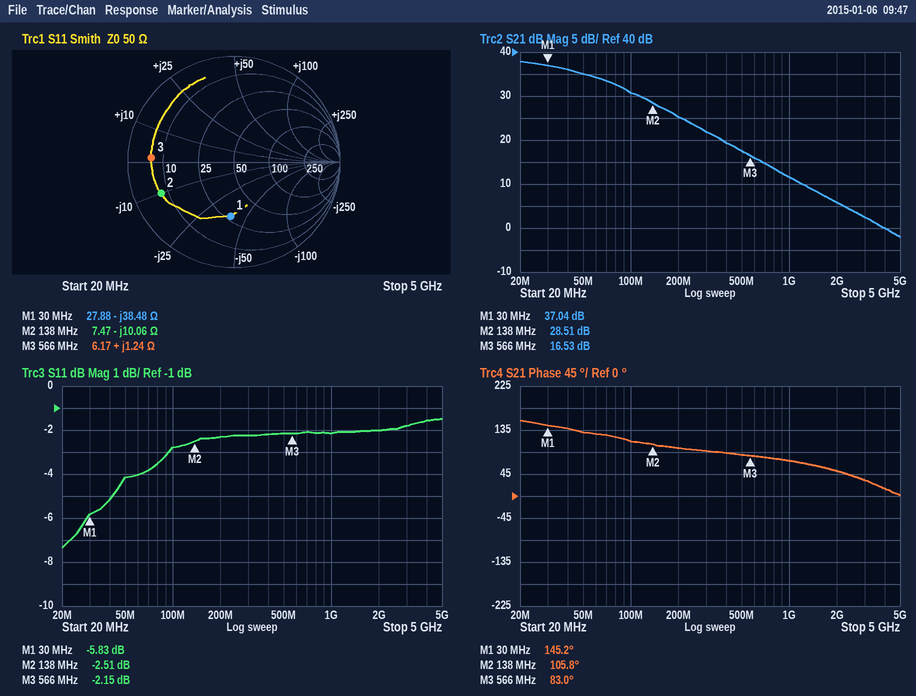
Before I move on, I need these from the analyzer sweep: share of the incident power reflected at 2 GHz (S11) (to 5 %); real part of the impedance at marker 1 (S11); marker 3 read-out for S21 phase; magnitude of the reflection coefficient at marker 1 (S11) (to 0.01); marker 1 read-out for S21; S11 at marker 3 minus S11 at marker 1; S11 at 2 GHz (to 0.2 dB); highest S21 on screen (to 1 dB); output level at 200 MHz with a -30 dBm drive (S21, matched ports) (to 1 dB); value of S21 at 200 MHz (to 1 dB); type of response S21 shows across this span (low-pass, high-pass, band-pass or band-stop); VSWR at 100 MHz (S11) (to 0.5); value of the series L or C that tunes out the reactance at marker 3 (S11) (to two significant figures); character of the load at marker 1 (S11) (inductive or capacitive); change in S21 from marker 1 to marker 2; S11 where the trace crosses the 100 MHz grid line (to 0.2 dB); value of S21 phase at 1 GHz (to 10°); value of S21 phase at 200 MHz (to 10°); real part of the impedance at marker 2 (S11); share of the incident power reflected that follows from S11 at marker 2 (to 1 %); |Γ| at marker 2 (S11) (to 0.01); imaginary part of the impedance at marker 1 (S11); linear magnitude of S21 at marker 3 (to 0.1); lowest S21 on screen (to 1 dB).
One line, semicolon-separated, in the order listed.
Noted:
65 %; 27.88 Ω; 83.0°; 0.51; 37.04 dB; 3.68 dB; -2.0 dB; 38 dB; -5 dBm; 25 dB; low-pass; 6.5; 230 pF; capacitive; -8.53 dB; -2.8 dB; 70°; 100°; 7.47 Ω; 56 %; 0.75; -38.48 Ω; 6.7; -2 dB
